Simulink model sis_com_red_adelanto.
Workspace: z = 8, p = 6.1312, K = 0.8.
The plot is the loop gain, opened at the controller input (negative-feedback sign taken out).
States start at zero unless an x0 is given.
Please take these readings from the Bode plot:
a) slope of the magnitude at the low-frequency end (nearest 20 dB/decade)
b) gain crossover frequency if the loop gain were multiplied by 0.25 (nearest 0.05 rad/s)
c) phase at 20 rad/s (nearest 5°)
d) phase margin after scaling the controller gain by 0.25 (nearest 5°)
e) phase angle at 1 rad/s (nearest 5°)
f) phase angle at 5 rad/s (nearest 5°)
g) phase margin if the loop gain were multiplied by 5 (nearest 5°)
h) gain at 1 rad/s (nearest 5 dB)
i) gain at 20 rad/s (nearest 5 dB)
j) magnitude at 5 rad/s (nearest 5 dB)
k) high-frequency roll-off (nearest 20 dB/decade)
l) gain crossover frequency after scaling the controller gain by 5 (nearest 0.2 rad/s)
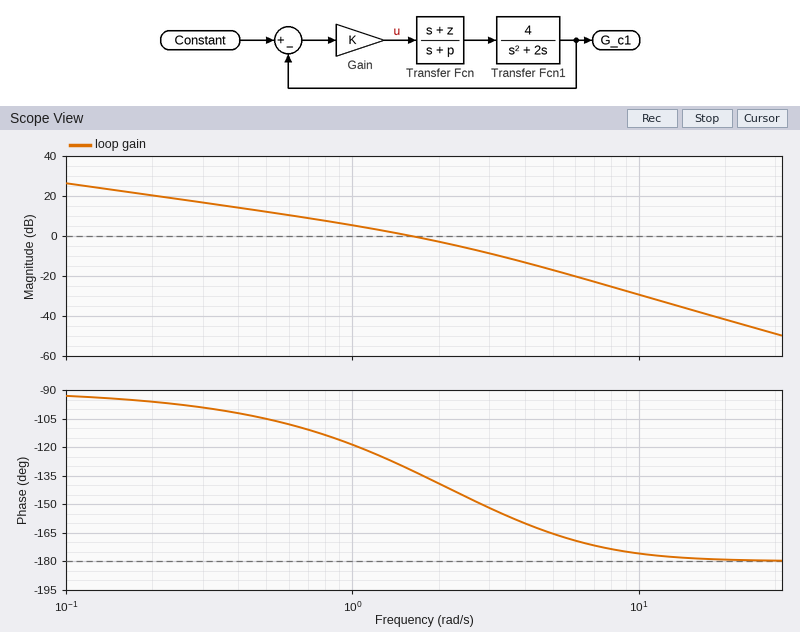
-20 dB/decade
0.50 rad/s
-180°
75°
-120°
-165°
20°
5 dB
-40 dB
-15 dB
-40 dB/decade
4.2 rad/s
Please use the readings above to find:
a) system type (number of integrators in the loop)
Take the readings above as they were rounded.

1
